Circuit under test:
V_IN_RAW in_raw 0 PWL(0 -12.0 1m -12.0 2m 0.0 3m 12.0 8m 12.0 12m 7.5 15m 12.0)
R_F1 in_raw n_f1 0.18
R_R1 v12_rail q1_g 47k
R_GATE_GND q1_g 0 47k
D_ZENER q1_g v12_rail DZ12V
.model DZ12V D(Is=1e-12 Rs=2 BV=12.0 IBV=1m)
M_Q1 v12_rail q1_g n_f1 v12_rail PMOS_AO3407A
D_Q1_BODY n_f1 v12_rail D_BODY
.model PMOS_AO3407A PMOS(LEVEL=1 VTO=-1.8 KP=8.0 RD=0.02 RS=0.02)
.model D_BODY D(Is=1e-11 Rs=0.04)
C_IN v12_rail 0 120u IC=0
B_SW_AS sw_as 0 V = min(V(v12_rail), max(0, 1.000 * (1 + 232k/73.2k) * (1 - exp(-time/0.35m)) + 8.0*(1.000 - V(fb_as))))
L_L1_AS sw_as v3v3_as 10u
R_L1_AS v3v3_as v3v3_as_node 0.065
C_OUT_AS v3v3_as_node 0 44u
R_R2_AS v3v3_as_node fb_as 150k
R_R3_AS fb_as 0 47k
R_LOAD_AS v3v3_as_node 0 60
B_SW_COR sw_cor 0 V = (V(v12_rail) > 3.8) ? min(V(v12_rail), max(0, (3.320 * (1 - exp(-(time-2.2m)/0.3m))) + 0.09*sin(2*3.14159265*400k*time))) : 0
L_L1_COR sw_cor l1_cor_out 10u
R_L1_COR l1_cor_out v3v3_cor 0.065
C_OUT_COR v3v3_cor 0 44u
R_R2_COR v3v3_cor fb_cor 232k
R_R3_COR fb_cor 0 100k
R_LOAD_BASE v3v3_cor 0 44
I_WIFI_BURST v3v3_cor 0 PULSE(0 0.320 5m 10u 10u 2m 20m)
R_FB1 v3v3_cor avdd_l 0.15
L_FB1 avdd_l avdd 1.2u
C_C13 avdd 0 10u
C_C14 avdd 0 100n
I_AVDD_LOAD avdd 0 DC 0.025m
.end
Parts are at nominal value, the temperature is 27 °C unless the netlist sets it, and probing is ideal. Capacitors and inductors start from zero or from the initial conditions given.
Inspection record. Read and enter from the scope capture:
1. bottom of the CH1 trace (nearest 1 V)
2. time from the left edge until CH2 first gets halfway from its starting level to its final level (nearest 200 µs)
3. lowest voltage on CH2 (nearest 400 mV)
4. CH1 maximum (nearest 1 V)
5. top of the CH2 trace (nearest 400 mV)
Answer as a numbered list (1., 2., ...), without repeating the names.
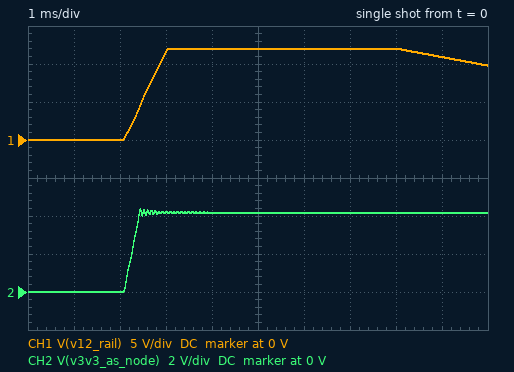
1. 0 V
2. 2.2 ms
3. 0 V
4. 12 V
5. 4.4 V
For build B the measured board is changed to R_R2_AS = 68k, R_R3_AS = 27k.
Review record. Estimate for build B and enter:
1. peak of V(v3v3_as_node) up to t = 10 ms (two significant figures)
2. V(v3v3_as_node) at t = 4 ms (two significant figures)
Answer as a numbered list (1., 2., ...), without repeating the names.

1. 3.9 V
2. 3.7 V
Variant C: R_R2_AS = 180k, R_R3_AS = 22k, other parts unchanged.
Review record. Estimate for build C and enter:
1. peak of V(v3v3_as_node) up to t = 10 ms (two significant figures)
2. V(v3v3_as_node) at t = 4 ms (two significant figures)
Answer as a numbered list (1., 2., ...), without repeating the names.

1. 6.7 V
2. 6.5 V
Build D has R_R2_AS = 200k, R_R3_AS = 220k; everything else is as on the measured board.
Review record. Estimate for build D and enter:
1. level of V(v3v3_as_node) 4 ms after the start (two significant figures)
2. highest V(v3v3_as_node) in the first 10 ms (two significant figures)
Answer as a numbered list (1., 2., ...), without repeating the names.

1. 2.3 V
2. 2.5 V
